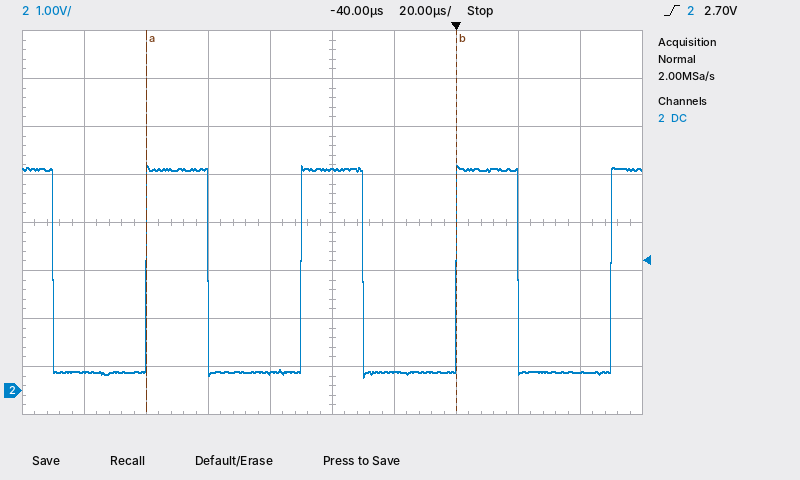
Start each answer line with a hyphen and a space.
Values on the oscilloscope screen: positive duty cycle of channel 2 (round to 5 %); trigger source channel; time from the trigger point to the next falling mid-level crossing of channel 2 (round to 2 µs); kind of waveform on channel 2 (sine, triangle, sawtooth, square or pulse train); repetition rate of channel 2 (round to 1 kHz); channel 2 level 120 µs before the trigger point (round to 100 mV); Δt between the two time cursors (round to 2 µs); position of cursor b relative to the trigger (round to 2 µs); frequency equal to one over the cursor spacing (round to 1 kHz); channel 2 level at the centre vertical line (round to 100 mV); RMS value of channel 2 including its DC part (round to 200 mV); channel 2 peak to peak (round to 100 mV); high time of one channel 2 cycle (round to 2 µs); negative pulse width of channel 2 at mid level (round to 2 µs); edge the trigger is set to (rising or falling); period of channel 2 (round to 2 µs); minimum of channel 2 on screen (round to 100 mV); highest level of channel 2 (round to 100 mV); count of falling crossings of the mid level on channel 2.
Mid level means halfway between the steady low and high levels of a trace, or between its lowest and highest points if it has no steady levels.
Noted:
- 40 %
- channel 2
- 20 µs
- pulse train
- 20 kHz
- 400 mV
- 100 µs
- 0 µs
- 10 kHz
- 4.6 V
- 3.0 V
- 4.4 V
- 20 µs
- 30 µs
- rising
- 50 µs
- 300 mV
- 4.7 V
- 4
